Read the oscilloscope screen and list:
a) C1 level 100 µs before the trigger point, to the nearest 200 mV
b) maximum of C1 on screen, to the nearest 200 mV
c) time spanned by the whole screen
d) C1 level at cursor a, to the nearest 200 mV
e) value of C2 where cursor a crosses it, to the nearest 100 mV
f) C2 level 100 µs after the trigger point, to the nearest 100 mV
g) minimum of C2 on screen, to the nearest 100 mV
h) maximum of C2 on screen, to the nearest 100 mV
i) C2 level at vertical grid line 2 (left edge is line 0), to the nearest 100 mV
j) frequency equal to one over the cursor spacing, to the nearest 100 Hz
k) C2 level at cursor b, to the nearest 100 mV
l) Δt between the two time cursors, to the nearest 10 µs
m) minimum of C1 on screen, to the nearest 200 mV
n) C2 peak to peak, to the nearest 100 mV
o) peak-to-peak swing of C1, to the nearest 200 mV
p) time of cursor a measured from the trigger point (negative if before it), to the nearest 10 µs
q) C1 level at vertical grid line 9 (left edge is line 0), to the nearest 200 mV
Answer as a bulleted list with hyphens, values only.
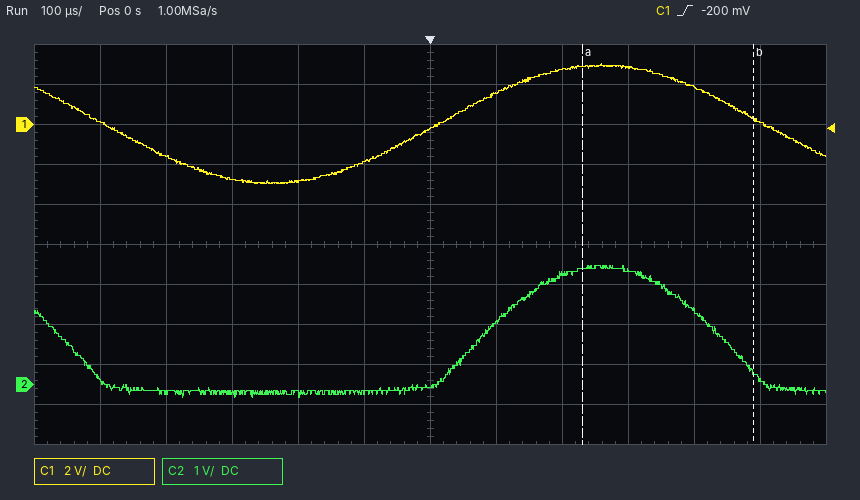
- -1.8 V
- 3.0 V
- 1.2 ms
- 3.0 V
- 2.9 V
- 1.5 V
- -300 mV
- 3.0 V
- -200 mV
- 3.8 kHz
- 300 mV
- 260 µs
- -3.0 V
- 3.3 V
- 6.0 V
- +230 µs
- 2.8 V
